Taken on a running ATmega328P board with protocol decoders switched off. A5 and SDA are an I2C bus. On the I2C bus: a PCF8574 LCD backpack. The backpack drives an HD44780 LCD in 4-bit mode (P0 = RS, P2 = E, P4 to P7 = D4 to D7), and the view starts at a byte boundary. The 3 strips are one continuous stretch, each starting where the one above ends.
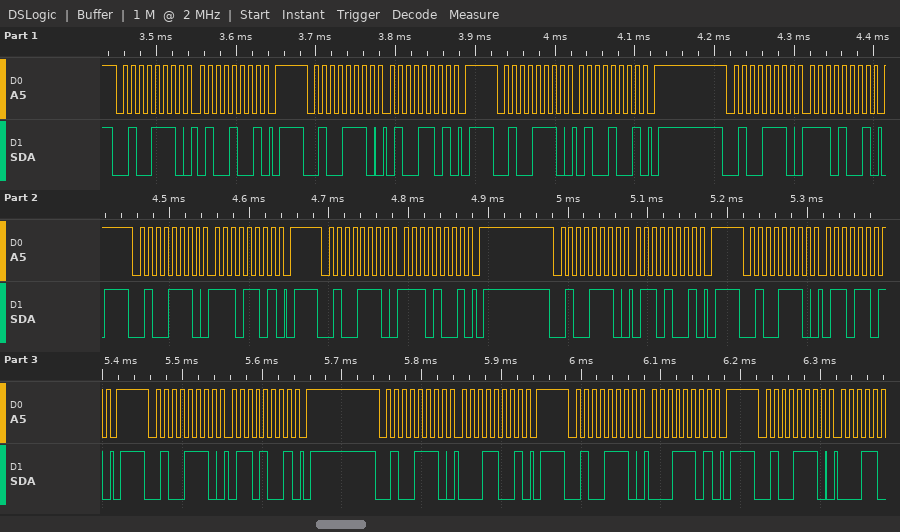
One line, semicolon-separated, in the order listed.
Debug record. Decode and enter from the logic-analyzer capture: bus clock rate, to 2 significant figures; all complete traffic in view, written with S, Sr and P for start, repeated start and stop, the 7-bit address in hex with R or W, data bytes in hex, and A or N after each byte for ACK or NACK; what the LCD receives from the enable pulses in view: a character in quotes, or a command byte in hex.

100 kHz; S 27W A 49 A P S 27W A 4D A P S 27W A 49 A P S 27W A E9 A P S 27W A ED A P S 27W A E9 A P S 27W A 69 A P S 27W A 6D A P S 27W A 69 A P S 27W A 19 A P S 27W A 1D A P S 27W A; 'N'
